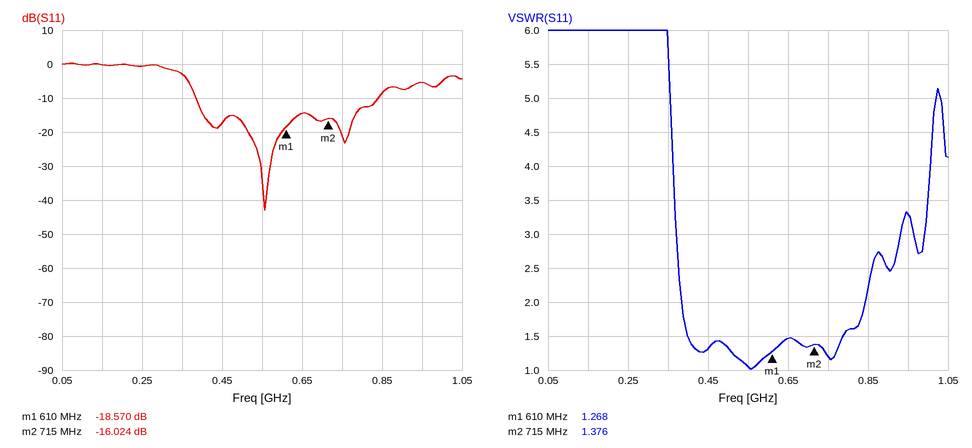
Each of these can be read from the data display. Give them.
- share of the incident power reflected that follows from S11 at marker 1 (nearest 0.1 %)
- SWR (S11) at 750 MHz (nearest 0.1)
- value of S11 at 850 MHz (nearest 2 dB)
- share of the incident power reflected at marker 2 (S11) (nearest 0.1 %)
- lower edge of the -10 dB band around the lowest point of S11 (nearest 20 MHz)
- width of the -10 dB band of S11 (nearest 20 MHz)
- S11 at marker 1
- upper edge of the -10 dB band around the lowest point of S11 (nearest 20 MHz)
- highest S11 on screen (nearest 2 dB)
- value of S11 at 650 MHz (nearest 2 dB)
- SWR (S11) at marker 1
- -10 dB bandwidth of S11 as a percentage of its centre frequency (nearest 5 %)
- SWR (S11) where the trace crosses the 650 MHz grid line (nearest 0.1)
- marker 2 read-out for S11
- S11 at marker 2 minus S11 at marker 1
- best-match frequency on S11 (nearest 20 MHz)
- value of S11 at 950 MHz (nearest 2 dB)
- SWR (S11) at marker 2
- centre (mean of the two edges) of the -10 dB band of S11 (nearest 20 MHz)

1.4 %
1.2
-8 dB
2.5 %
380 MHz
460 MHz
-18.570 dB
840 MHz
0 dB
-14 dB
1.268
75 %
1.5
-16.024 dB
2.546 dB
560 MHz
-6 dB
1.376
620 MHz
